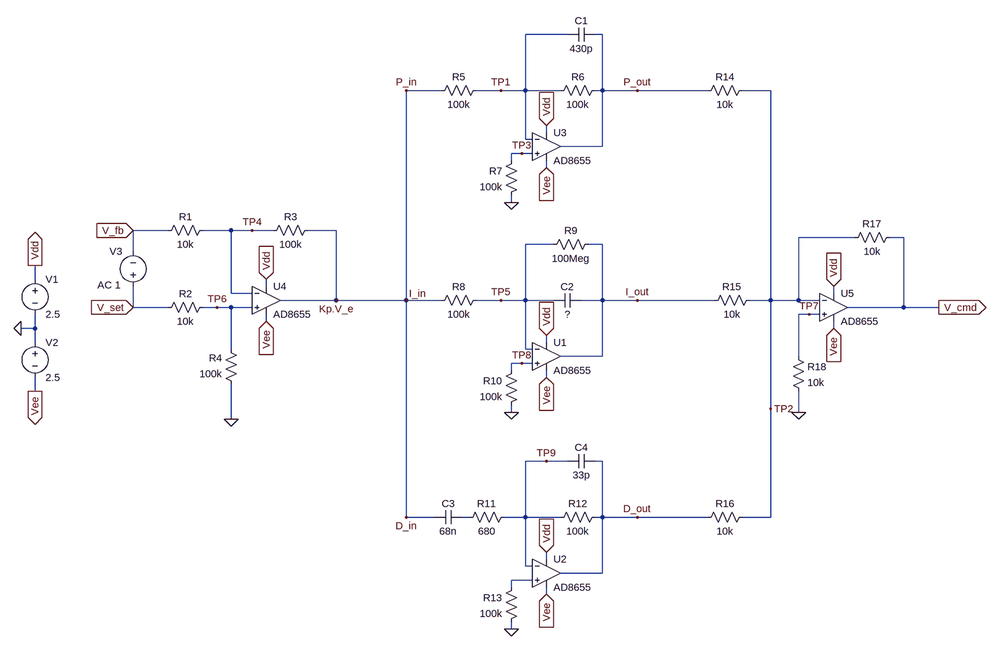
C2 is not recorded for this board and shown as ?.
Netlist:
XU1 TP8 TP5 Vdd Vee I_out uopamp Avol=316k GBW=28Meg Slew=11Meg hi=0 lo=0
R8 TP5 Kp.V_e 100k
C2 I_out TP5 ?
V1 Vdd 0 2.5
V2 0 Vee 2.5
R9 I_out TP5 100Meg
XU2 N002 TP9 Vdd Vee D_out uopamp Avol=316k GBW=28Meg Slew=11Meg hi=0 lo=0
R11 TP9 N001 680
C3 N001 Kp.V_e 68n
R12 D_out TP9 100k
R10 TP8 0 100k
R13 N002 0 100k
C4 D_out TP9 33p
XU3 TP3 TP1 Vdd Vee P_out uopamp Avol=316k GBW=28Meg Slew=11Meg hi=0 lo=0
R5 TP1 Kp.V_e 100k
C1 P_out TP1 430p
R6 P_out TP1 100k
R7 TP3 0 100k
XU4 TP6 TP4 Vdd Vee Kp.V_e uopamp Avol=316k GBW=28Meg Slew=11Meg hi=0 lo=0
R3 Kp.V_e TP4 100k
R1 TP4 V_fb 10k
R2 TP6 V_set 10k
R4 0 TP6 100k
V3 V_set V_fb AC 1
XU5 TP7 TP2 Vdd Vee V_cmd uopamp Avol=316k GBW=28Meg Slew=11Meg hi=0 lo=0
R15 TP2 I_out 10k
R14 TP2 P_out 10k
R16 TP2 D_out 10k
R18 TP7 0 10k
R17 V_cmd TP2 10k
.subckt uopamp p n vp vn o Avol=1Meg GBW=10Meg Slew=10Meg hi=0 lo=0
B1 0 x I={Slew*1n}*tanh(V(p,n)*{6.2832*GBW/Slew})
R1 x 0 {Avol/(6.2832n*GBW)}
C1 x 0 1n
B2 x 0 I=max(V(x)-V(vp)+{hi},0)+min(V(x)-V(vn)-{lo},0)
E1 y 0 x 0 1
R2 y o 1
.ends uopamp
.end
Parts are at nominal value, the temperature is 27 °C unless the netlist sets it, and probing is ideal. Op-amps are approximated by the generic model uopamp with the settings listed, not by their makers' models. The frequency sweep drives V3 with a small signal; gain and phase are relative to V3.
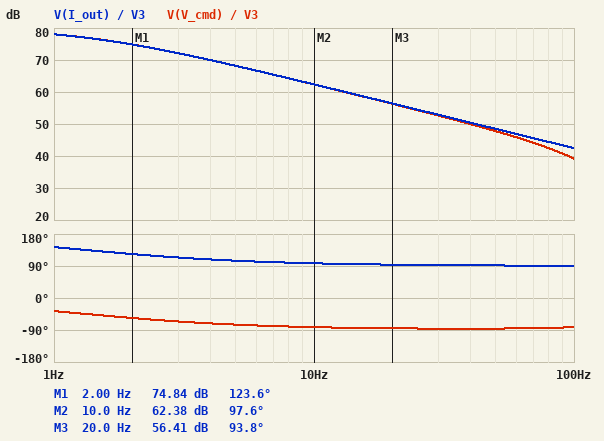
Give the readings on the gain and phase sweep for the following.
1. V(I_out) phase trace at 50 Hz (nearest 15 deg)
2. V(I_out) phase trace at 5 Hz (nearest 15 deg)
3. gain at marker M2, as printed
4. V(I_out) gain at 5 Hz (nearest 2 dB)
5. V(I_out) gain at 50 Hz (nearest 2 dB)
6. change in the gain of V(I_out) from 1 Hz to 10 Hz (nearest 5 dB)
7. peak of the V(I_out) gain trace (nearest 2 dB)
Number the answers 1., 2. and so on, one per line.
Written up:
1. 90 deg
2. 105 deg
3. 62.38 dB
4. 68 dB
5. 48 dB
6. -15 dB
7. 78 dB
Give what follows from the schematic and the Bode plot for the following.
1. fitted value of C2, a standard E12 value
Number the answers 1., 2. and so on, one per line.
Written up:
1. 1.2 nF
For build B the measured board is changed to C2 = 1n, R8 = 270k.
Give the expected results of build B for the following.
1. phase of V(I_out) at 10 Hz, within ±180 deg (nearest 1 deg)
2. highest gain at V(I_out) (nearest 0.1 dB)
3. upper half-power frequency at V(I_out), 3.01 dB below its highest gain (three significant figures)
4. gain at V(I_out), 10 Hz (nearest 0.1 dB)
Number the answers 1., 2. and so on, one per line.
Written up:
1. 99 deg
2. 71.4 dB
3. 1.59 Hz
4. 55.3 dB
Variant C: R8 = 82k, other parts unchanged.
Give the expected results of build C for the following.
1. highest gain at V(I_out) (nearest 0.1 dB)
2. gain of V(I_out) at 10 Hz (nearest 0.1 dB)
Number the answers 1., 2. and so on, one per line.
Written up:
1. 81.7 dB
2. 64.1 dB
